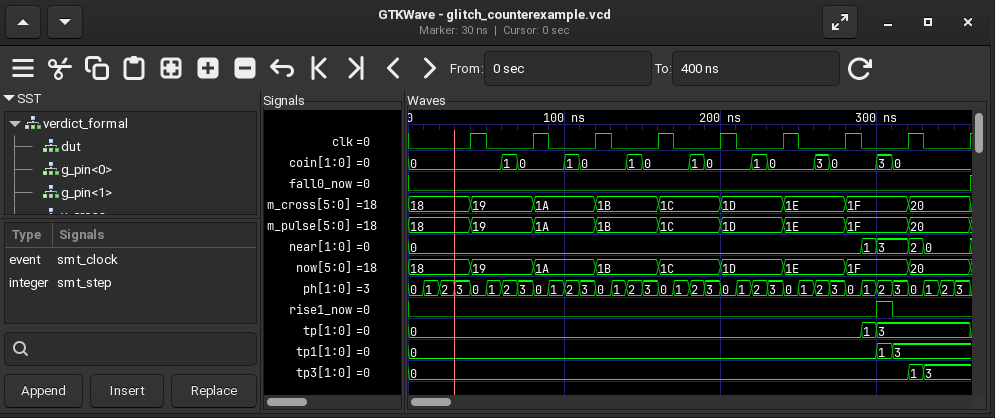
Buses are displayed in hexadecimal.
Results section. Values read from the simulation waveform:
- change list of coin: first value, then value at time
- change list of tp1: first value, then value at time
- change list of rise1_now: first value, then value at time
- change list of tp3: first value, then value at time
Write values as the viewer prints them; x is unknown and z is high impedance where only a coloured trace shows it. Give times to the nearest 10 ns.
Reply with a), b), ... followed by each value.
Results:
a) 0, 1 at 60 ns, 0 at 70 ns, 1 at 100 ns, 0 at 110 ns, 1 at 140 ns, 0 at 150 ns, 1 at 180 ns, 0 at 190 ns, 1 at 220 ns, 0 at 230 ns, 3 at 260 ns, 0 at 270 ns, 3 at 300 ns, 0 at 310 ns
b) 0, 1 at 300 ns, 3 at 310 ns
c) 0, 1 at 300 ns, 0 at 310 ns
d) 0, 1 at 320 ns, 3 at 330 ns
